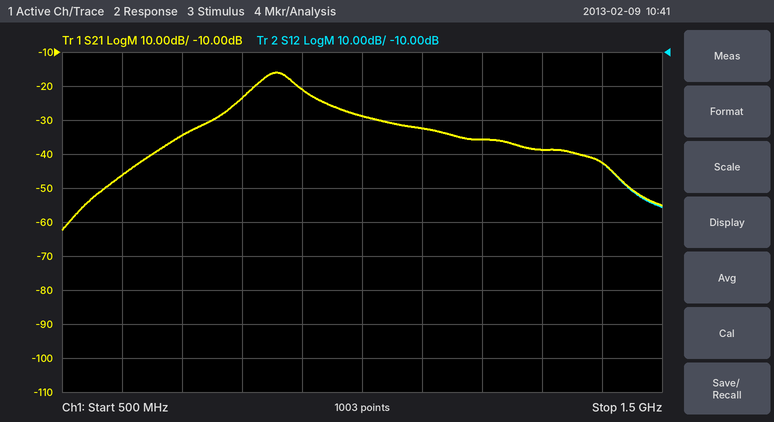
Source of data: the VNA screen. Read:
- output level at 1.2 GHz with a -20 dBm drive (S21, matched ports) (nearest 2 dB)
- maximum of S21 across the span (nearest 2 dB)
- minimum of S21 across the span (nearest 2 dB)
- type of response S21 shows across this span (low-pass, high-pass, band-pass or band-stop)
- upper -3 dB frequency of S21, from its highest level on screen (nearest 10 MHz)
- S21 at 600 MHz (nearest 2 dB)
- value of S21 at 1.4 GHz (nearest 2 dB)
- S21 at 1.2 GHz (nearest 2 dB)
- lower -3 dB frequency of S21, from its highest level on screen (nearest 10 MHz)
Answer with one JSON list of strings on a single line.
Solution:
["-56 dBm", "-16 dB", "-62 dB", "band-pass", "890 MHz", "-46 dB", "-42 dB", "-36 dB", "830 MHz"]
